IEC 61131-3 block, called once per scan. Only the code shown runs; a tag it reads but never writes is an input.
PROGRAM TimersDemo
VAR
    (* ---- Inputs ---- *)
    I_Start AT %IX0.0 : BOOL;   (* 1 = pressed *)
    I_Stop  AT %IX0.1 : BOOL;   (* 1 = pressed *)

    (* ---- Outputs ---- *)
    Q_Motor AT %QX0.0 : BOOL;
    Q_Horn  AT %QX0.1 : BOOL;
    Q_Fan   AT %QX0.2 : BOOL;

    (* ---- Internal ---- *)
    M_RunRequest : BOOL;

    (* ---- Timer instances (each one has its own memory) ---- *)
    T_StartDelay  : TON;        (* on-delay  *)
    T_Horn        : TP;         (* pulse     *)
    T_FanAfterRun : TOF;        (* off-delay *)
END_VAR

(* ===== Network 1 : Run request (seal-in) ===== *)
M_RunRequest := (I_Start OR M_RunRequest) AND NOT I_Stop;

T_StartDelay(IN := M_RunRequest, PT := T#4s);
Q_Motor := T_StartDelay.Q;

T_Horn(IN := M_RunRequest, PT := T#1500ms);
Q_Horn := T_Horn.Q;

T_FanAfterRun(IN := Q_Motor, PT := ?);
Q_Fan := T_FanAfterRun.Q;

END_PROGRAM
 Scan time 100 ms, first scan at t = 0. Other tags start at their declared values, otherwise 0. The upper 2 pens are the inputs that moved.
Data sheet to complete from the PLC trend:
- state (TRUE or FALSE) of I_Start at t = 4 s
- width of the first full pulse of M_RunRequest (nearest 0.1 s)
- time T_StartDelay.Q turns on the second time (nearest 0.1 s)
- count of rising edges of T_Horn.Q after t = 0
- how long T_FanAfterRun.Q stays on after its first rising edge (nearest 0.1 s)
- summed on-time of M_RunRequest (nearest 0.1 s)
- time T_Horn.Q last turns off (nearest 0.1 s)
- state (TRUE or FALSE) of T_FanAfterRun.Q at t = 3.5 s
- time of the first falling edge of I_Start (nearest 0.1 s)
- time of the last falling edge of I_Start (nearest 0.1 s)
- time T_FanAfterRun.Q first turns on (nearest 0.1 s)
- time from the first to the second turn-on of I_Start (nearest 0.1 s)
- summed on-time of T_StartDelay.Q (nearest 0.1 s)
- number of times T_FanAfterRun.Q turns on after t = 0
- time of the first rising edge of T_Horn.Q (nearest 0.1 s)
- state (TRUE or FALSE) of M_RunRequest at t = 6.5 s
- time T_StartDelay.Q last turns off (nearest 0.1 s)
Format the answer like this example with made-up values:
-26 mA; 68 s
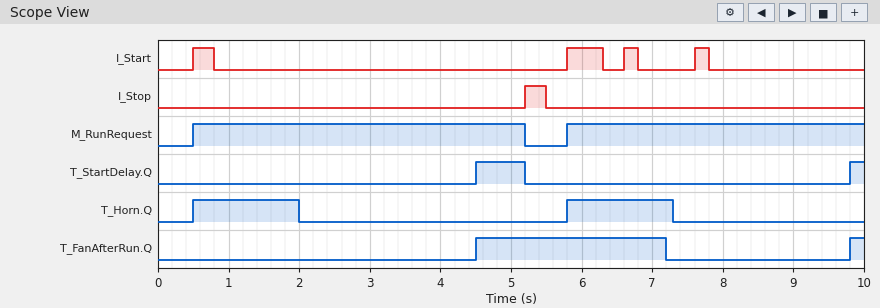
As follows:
FALSE; 4.7 s; 9.8 s; 2; 2.7 s; 8.9 s; 7.3 s; FALSE; 0.8 s; 7.8 s; 4.5 s; 5.3 s; 0.9 s; 2; 0.5 s; TRUE; 5.2 s
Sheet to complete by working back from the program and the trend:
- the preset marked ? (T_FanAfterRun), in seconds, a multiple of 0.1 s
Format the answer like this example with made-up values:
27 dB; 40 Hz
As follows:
2.0 s
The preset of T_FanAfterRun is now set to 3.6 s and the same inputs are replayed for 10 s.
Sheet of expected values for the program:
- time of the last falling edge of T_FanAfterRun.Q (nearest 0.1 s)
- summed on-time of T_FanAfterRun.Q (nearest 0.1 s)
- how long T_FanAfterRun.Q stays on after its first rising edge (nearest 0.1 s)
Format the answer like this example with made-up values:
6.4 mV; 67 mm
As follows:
8.8 s; 4.5 s; 4.3 s
